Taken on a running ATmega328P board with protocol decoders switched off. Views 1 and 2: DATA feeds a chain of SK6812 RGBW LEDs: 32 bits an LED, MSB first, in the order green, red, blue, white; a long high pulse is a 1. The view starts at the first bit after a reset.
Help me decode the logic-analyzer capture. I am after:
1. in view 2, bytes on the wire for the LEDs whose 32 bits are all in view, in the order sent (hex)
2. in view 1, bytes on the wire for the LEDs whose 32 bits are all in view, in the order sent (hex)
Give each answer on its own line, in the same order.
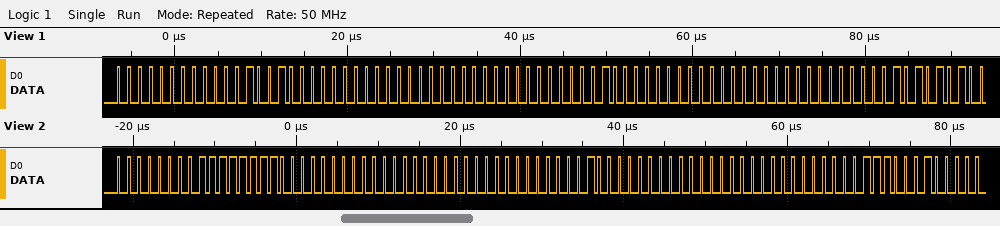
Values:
00 FF 00 00 00 02 00 00
00 09 00 00 00 04 00 00
